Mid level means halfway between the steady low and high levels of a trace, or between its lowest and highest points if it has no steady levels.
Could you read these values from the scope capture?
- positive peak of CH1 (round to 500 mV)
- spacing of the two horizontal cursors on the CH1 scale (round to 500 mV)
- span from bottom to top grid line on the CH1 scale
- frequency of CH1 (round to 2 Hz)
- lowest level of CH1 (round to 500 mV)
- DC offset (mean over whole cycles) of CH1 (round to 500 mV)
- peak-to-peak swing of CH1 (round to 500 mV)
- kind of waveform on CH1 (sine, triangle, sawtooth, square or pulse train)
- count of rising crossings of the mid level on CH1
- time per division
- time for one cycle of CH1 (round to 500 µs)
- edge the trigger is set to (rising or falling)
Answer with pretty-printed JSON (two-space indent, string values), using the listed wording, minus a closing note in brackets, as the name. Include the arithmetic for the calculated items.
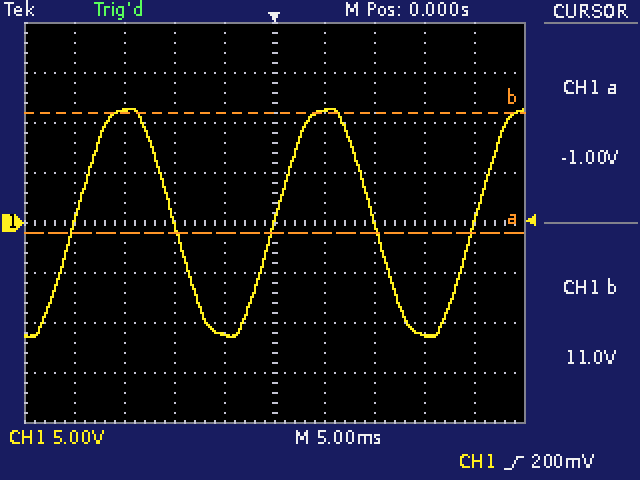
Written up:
{
  "positive peak of CH1": "11.5 V",
  "spacing of the two horizontal cursors on the CH1 scale": "12.0 V",
  "span from bottom to top grid line on the CH1 scale": "40 V",
  "frequency of CH1": "1 / 20.0 ms ≈ 50 Hz",
  "lowest level of CH1": "-11.5 V",
  "DC offset (mean over whole cycles) of CH1": "(11.5 V + (-11.5 V)) / 2 ≈ 0.0 V",
  "peak-to-peak swing of CH1": "11.5 V − (-11.5 V) = 23.0 V",
  "kind of waveform on CH1": "sine",
  "count of rising crossings of the mid level on CH1": "3",
  "time per division": "5 ms",
  "time for one cycle of CH1": "20.0 ms",
  "edge the trigger is set to": "rising"
}
